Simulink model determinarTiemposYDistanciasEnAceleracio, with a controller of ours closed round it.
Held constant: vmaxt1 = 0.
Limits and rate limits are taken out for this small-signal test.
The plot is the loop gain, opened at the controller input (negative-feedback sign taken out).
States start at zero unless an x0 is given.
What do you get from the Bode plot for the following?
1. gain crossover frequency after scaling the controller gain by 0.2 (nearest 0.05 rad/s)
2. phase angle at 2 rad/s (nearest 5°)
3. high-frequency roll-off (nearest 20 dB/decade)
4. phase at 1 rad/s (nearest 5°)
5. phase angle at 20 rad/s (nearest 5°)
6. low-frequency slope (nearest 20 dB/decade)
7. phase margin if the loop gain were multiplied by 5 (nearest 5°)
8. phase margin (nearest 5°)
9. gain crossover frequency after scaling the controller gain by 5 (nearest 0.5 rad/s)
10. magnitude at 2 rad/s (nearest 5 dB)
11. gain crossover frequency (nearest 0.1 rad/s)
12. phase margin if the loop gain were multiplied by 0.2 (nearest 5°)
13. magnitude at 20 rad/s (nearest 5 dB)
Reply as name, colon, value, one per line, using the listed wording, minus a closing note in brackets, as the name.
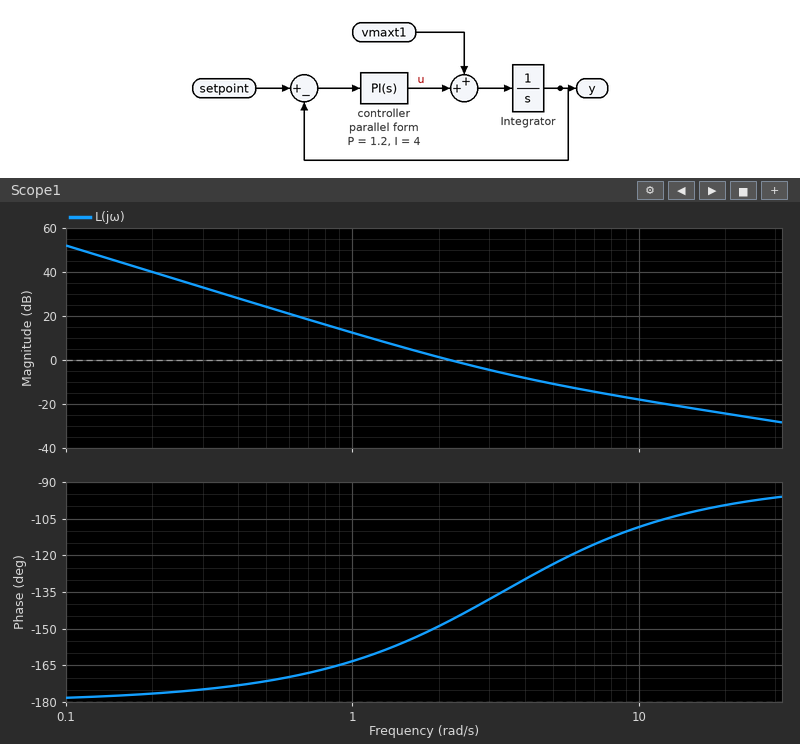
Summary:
gain crossover frequency after scaling the controller gain by 0.2: 0.90 rad/s
phase angle at 2 rad/s: -150°
high-frequency roll-off: -20 dB/decade
phase at 1 rad/s: -165°
phase angle at 20 rad/s: -100°
low-frequency slope: -40 dB/decade
phase margin if the loop gain were multiplied by 5: 65°
phase margin: 35°
gain crossover frequency after scaling the controller gain by 5: 6.5 rad/s
magnitude at 2 rad/s: 0 dB
gain crossover frequency: 2.2 rad/s
phase margin if the loop gain were multiplied by 0.2: 15°
magnitude at 20 rad/s: -25 dB
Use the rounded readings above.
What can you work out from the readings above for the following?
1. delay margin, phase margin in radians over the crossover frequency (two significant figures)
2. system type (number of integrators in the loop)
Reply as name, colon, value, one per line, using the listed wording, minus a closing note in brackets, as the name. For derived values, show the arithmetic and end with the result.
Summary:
delay margin, phase margin in radians over the crossover frequency: 35 × π / 180 / 2.2 = 0.28 s
system type: 2
